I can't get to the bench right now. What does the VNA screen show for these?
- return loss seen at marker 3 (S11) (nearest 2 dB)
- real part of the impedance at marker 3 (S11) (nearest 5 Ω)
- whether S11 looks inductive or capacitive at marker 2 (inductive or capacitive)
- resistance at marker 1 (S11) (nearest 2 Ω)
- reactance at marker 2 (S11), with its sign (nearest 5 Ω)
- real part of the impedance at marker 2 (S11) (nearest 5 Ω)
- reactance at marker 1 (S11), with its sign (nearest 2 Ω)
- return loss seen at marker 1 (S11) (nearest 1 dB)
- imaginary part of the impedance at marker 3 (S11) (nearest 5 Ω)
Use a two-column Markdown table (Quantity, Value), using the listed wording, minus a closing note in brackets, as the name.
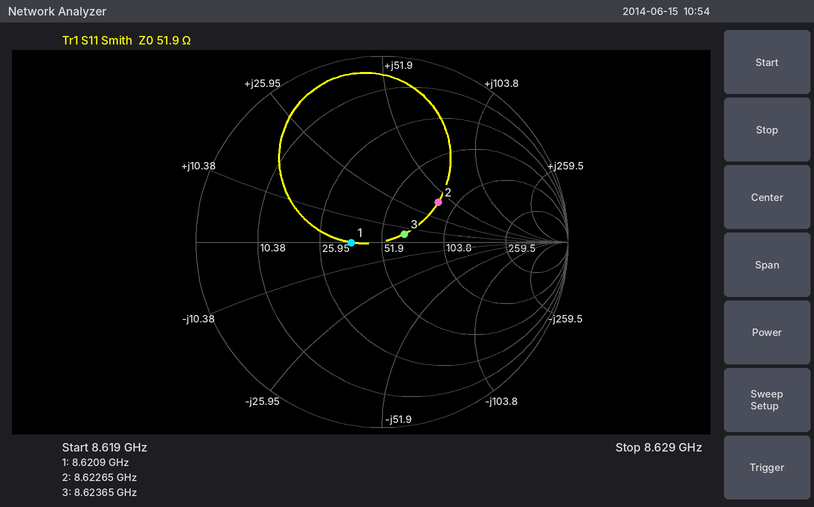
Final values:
| Quantity | Value |
|---|---|
| return loss seen at marker 3 (S11) | 18 dB |
| real part of the impedance at marker 3 (S11) | 65 Ω |
| whether S11 looks inductive or capacitive at marker 2 | inductive |
| resistance at marker 1 (S11) | 38 Ω |
| reactance at marker 2 (S11), with its sign | +40 Ω |
| real part of the impedance at marker 2 (S11) | 85 Ω |
| reactance at marker 1 (S11), with its sign | 0 Ω |
| return loss seen at marker 1 (S11) | 16 dB |
| imaginary part of the impedance at marker 3 (S11) | +5 Ω |
